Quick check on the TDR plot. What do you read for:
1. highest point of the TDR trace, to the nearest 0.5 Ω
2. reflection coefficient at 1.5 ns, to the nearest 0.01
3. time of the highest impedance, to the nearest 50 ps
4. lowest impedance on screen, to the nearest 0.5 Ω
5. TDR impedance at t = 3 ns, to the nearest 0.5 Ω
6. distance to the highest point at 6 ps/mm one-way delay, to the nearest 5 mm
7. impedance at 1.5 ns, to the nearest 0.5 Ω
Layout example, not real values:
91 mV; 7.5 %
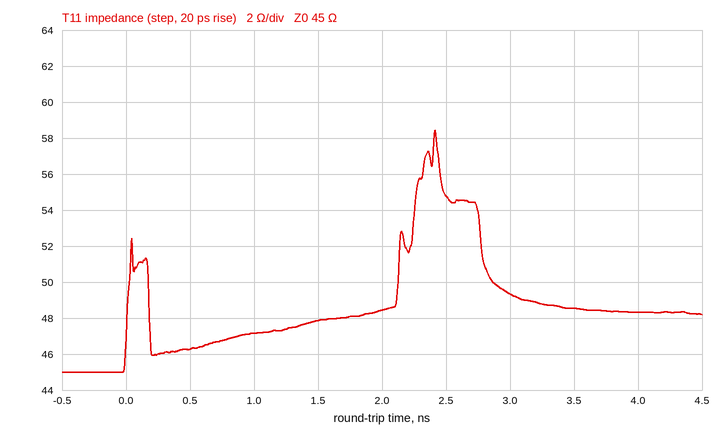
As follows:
58.5 Ω; +0.03; 2.40 ns; 45.0 Ω; 49.5 Ω; 200 mm; 48.0 Ω
